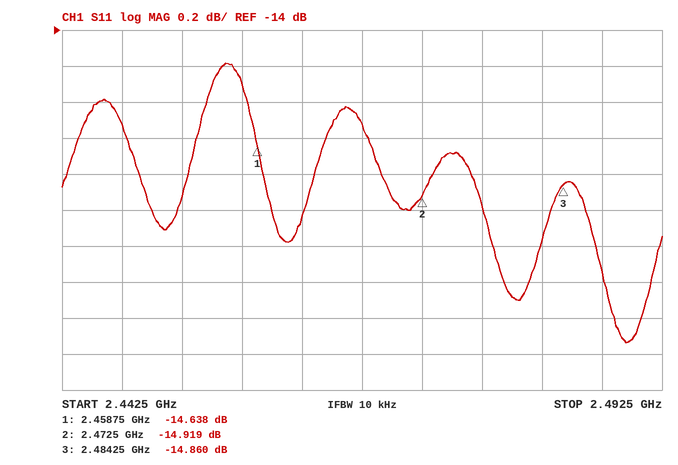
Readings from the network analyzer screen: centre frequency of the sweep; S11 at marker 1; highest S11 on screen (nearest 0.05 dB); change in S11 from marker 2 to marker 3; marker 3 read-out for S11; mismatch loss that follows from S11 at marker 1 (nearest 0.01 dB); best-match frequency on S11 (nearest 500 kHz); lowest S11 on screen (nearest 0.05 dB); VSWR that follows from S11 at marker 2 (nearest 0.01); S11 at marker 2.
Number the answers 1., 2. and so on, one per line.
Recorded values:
1. 2.4675 GHz
2. -14.638 dB
3. -14.20 dB
4. 0.059 dB
5. -14.860 dB
6. 0.15 dB
7. 2.4895 GHz
8. -15.75 dB
9. 1.44
10. -14.919 dB
